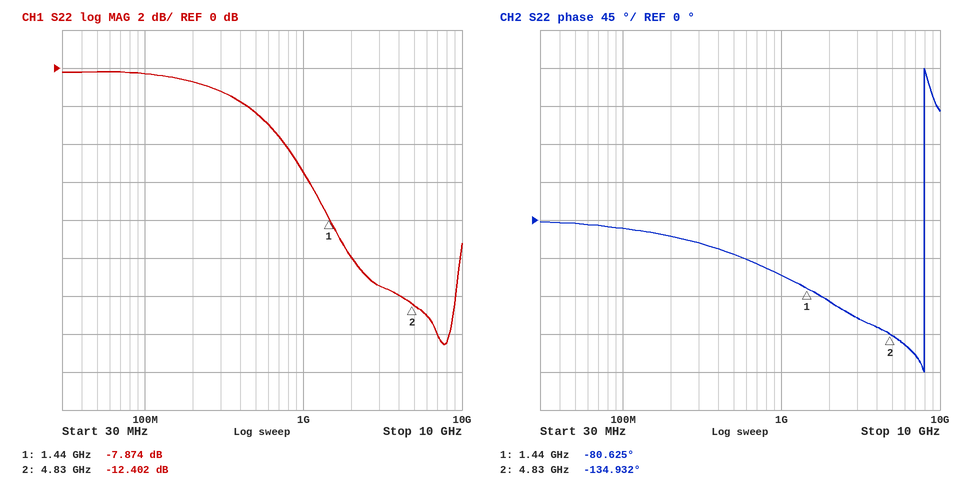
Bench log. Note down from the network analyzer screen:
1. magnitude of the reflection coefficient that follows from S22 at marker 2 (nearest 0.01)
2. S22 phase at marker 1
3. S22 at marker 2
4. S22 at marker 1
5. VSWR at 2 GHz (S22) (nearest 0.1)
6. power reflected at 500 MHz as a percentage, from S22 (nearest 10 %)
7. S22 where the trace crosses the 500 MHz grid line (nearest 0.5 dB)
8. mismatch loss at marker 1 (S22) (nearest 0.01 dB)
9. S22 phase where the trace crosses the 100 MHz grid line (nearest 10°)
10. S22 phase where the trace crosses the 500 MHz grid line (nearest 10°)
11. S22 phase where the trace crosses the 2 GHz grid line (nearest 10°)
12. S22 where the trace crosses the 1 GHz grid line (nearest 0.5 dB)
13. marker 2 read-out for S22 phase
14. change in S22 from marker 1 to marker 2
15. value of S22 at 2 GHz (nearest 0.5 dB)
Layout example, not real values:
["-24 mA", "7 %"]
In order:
["0.24", "-80.625°", "-12.402 dB", "-7.874 dB", "1.9", "60 %", "-2.5 dB", "0.77 dB", "-10°", "-40°", "-100°", "-5.5 dB", "-134.932°", "-4.528 dB", "-10.0 dB"]
